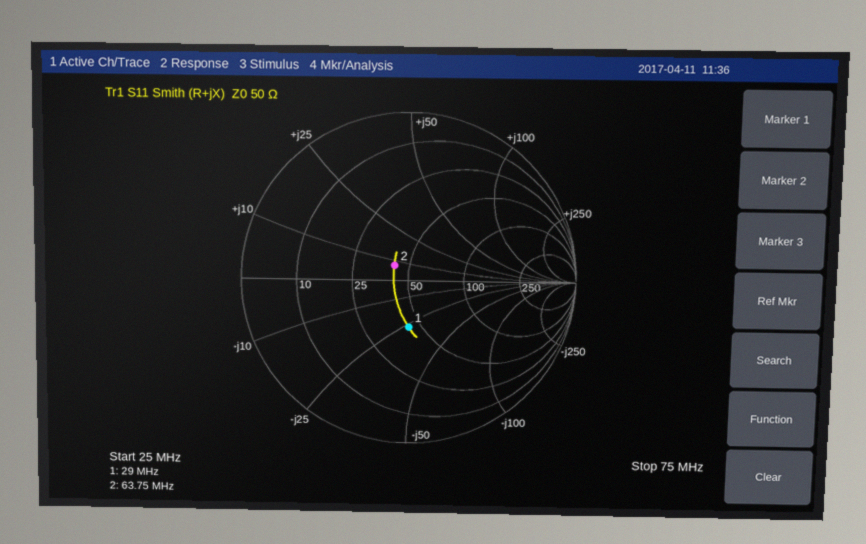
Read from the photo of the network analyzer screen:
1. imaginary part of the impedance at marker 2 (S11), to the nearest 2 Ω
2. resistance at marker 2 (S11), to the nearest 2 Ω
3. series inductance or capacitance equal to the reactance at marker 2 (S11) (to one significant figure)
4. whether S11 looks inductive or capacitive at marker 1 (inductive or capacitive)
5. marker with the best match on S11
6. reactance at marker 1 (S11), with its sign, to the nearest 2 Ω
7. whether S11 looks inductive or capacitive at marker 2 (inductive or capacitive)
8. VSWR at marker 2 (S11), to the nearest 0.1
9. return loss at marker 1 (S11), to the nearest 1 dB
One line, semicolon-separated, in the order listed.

+8 Ω; 42 Ω; 20 nH; capacitive; marker 2; -26 Ω; inductive; 1.3; 11 dB
